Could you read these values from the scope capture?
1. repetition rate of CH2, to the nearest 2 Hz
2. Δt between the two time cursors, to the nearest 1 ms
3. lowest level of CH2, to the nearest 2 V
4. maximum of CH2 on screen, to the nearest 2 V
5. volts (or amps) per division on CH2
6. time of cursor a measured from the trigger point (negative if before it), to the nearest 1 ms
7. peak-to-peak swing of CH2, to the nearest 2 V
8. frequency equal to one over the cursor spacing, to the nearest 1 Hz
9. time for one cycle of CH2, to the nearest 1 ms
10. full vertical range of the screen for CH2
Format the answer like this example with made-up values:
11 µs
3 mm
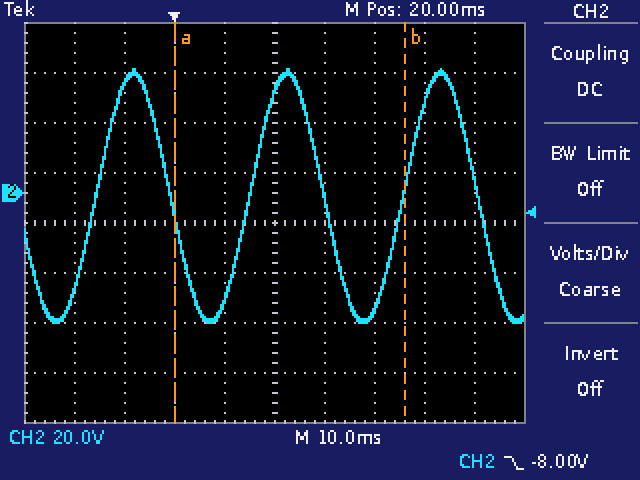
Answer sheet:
32 Hz
46 ms
-52 V
50 V
20 V
0 ms
102 V
22 Hz
31 ms
160 V
